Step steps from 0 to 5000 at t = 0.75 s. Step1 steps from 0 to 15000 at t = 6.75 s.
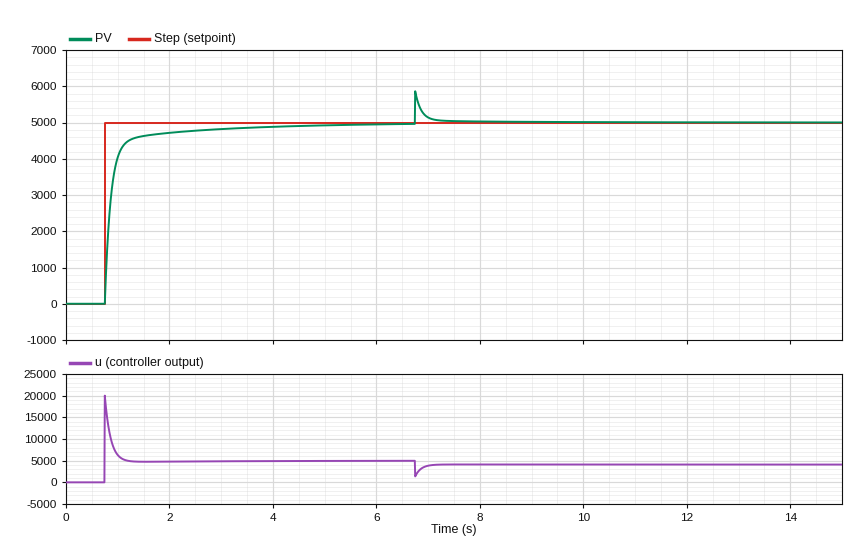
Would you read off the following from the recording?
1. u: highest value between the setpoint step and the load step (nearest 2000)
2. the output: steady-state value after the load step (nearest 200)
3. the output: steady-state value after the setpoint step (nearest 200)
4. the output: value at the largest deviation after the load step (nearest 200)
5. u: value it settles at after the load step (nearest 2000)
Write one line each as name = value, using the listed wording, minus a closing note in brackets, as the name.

u: highest value between the setpoint step and the load step = 20000
the output: steady-state value after the load step = 5000
the output: steady-state value after the setpoint step = 5000
the output: value at the largest deviation after the load step = 5800
u: value it settles at after the load step = 4000
